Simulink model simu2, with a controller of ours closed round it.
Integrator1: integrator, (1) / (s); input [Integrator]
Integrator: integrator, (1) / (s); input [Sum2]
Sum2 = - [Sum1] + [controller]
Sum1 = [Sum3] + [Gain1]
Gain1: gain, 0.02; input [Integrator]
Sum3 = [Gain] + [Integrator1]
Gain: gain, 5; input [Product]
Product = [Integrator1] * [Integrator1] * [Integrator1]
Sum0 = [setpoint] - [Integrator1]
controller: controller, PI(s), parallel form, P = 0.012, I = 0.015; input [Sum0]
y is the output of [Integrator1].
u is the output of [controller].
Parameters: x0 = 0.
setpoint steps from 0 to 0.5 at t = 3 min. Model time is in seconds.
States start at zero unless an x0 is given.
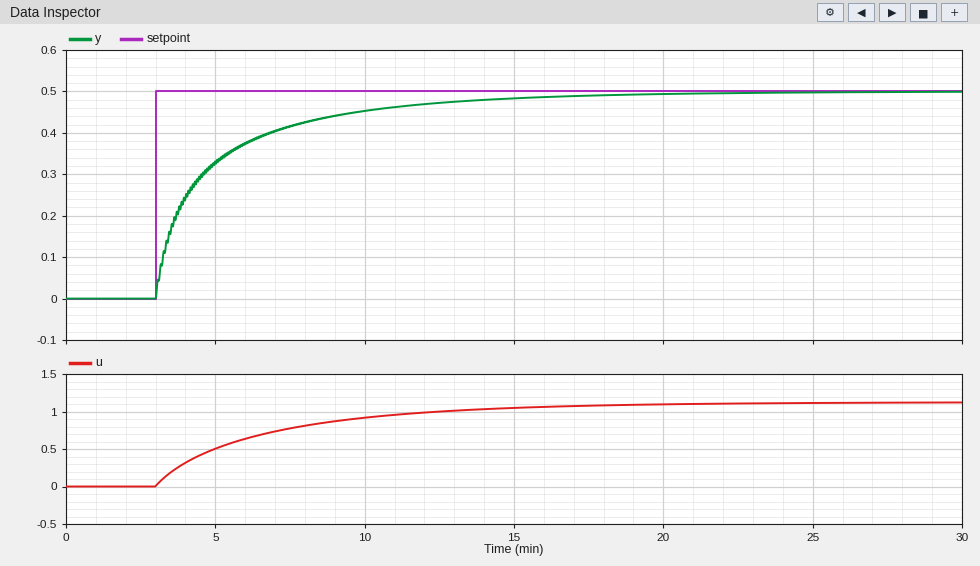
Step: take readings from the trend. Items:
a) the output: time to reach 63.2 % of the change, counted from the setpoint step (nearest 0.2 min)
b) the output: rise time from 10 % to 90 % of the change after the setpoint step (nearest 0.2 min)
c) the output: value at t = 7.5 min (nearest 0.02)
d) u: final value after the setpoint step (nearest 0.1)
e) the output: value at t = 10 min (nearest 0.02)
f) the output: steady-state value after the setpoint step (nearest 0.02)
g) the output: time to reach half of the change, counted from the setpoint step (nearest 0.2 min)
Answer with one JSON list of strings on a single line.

["1.8 min", "6.6 min", "0.42", "1.1", "0.46", "0.50", "1.0 min"]
